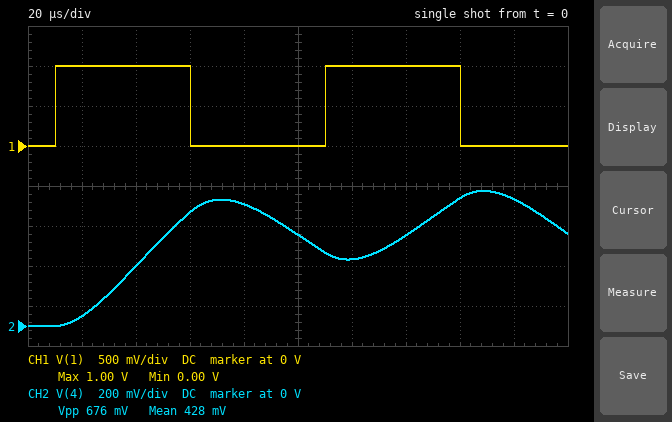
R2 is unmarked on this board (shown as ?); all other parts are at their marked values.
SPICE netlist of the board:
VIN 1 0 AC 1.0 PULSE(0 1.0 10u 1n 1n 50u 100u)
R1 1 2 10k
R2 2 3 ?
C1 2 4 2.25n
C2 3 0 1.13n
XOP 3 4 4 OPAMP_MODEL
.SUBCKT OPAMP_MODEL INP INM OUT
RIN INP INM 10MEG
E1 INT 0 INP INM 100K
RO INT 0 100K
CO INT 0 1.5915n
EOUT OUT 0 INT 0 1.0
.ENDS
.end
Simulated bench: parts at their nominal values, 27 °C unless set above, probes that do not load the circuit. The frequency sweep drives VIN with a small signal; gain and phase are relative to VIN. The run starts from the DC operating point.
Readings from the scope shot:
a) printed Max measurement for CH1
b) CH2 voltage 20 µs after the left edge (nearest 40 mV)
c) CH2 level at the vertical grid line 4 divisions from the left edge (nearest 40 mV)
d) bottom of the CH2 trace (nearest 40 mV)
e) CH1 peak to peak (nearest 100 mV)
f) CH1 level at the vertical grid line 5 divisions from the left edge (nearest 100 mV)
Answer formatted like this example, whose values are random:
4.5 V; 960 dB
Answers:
1.00 V; 40 mV; 600 mV; 0 V; 1.0 V; 0 V
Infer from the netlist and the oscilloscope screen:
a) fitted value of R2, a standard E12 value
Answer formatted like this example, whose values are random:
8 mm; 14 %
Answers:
33 kΩ
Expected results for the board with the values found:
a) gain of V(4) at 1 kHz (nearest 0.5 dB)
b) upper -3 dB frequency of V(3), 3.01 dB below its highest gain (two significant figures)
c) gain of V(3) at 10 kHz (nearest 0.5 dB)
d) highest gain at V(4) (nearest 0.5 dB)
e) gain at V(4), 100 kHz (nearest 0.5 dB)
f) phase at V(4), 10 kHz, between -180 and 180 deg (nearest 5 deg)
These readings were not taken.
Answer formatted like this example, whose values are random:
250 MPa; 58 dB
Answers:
0 dB; 4.5 kHz; -11.5 dB; 0 dB; -50.5 dB; -125 deg
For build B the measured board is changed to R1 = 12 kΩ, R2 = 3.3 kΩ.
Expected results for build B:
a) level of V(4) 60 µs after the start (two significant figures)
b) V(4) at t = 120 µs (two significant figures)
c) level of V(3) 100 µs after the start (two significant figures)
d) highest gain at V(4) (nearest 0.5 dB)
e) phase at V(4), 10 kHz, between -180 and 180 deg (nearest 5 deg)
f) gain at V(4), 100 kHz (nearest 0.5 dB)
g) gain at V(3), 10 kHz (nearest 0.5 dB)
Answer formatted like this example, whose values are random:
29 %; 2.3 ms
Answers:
1.0 V; 280 mV; 36 mV; 0 dB; -60 deg; -32.0 dB; -2.0 dB
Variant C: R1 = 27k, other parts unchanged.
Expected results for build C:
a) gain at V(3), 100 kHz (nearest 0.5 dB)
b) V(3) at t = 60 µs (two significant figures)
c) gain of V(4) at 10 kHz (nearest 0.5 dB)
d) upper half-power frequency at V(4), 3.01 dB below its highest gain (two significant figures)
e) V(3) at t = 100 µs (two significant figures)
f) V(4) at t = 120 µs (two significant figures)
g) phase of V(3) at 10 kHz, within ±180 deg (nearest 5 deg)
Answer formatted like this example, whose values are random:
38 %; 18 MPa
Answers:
-59.0 dB; 330 mV; -19.0 dB; 3.3 kHz; 450 mV; 410 mV; -150 deg
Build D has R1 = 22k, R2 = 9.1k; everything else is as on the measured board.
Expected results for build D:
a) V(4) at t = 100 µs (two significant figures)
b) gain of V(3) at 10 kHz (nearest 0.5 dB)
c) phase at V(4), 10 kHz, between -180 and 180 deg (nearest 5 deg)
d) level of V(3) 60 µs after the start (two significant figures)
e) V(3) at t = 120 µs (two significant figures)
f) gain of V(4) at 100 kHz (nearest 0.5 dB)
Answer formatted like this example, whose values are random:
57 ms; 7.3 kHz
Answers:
390 mV; -7.5 dB; -115 deg; 750 mV; 240 mV; -46.0 dB
